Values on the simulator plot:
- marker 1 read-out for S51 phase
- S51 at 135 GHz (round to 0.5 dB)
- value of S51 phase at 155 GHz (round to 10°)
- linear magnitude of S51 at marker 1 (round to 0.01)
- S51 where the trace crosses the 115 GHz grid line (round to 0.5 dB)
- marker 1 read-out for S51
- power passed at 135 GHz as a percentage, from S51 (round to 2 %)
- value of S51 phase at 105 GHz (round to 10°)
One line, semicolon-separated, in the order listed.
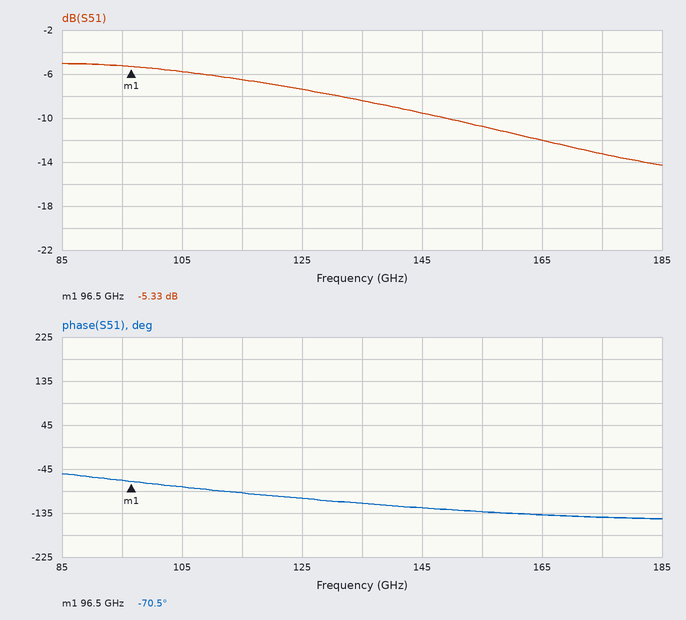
-70.5°; -8.5 dB; -130°; 0.54; -6.5 dB; -5.33 dB; 14 %; -80°
